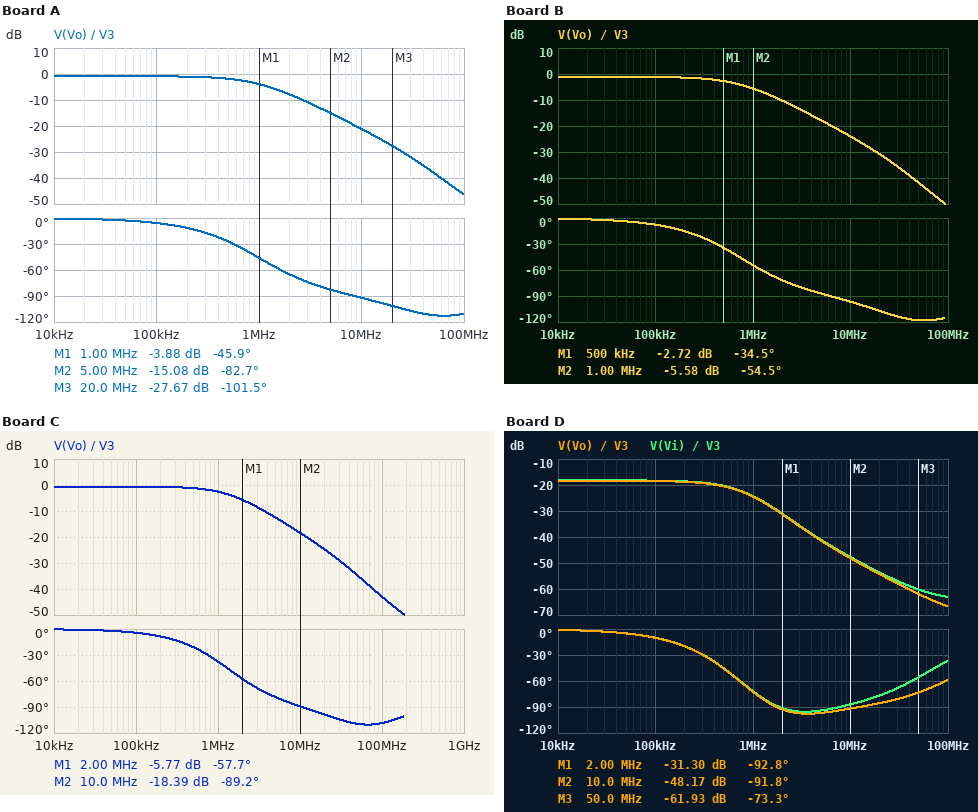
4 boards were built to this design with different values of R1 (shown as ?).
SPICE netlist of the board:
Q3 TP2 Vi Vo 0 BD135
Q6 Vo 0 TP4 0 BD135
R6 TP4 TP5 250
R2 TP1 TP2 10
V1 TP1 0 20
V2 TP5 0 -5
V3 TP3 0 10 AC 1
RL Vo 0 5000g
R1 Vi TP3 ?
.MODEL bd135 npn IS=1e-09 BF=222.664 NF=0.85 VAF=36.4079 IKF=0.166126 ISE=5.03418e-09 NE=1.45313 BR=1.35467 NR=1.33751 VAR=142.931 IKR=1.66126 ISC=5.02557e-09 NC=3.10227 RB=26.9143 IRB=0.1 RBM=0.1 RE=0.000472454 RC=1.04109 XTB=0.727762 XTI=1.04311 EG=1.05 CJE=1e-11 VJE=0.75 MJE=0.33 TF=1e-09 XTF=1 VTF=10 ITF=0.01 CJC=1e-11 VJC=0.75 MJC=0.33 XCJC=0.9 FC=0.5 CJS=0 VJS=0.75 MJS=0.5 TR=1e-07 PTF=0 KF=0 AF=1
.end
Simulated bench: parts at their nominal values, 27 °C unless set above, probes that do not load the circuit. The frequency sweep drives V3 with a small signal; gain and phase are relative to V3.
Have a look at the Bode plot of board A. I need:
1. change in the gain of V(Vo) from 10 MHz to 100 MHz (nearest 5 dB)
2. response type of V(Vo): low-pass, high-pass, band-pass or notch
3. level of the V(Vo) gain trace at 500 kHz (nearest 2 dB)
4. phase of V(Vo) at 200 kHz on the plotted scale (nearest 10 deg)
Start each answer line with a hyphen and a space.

- -25 dB
- low-pass
- -2 dB
- -10 deg
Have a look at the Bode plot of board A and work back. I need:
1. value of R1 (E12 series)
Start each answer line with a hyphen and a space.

- 47 kΩ
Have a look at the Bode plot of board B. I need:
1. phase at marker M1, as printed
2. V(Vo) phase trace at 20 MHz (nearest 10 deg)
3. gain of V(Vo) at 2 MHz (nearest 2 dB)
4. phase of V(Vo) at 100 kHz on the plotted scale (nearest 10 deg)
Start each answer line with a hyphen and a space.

- -34.5 deg
- -110 deg
- -10 dB
- -10 deg
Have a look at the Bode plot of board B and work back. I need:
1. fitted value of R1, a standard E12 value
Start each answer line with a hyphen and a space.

- 68 kΩ
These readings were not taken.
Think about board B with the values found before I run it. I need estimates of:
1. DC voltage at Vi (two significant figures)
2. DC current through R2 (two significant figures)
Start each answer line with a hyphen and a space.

- 1.1 V
- 18 mA
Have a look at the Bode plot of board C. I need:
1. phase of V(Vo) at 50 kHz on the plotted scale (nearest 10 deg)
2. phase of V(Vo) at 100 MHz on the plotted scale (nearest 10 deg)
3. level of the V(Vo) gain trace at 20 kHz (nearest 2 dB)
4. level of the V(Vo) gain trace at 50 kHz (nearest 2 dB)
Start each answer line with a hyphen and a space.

- 0 deg
- -110 deg
- 0 dB
- 0 dB
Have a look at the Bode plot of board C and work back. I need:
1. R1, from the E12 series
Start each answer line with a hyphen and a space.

- 33 kΩ
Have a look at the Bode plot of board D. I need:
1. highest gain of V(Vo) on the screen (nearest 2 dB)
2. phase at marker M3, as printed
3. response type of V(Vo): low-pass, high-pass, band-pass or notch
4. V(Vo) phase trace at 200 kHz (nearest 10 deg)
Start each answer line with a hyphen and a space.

- -18 dB
- -73.3 deg
- low-pass
- -20 deg
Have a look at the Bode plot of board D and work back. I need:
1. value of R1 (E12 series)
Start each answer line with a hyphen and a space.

- 82 kΩ
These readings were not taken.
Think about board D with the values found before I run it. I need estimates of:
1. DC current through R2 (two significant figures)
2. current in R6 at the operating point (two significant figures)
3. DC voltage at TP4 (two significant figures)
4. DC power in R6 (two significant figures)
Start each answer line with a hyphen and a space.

- 17 mA
- 18 mA
- -400 mV
- 85 mW
